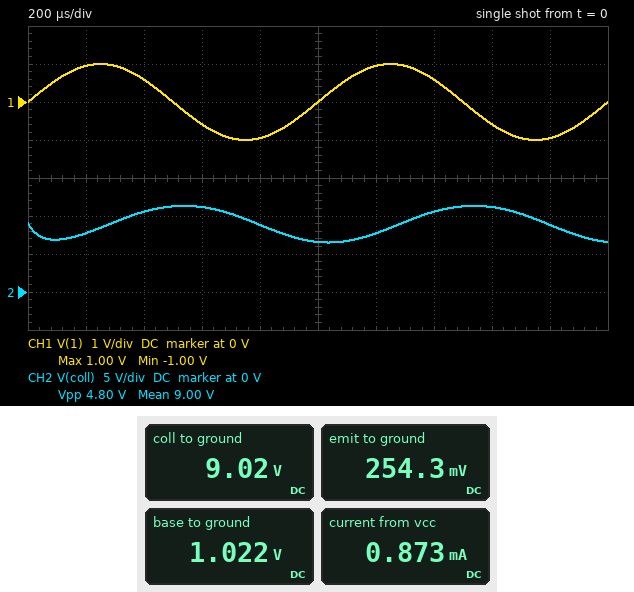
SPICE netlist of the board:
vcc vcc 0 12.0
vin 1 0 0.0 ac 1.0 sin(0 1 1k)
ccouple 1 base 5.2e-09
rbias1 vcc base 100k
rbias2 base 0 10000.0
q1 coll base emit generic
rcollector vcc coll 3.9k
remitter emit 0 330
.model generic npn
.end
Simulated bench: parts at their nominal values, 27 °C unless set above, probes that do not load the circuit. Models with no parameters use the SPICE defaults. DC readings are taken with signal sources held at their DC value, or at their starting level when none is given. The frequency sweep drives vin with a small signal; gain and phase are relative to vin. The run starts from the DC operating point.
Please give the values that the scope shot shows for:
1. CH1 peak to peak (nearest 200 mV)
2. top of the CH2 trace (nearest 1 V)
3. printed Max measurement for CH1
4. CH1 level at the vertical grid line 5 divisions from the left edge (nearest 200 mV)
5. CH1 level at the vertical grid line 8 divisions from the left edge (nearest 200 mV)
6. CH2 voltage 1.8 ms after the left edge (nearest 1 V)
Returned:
2.0 V
11 V
1.00 V
0 V
-600 mV
9 V
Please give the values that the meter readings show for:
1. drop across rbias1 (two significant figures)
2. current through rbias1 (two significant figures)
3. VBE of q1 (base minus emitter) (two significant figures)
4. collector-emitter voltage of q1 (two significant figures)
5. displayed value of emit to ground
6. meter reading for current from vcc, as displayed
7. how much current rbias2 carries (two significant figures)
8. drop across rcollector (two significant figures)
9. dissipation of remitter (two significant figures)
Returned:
11 V
110 µA
770 mV
8.8 V
254.3 mV
0.873 mA
100 µA
3.0 V
200 µW
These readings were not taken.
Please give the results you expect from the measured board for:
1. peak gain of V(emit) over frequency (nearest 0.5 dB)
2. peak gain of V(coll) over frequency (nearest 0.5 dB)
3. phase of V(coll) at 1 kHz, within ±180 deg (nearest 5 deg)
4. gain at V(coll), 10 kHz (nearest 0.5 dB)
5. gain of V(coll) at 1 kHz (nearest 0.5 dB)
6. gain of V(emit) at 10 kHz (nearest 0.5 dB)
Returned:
-1.0 dB
20.5 dB
-105 deg
20.0 dB
8.0 dB
-1.5 dB
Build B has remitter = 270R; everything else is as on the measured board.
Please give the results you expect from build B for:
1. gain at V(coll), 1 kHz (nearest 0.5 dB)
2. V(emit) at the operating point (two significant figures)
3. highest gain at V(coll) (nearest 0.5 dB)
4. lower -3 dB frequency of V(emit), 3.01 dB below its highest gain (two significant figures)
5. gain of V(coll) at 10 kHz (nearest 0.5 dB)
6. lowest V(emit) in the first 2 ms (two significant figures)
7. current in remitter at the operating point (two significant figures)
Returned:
9.0 dB
240 mV
22.0 dB
4.4 kHz
21.5 dB
53 mV
890 µA
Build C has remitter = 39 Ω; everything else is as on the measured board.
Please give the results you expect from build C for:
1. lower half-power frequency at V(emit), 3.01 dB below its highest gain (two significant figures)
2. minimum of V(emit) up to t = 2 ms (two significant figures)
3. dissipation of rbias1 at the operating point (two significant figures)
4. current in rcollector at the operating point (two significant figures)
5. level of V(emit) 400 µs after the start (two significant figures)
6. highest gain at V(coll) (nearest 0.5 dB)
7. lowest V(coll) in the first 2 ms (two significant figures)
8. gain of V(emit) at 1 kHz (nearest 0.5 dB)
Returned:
9.4 kHz
15 mV
1.2 mW
2.3 mA
32 mV
37.5 dB
250 mV
-21.5 dB
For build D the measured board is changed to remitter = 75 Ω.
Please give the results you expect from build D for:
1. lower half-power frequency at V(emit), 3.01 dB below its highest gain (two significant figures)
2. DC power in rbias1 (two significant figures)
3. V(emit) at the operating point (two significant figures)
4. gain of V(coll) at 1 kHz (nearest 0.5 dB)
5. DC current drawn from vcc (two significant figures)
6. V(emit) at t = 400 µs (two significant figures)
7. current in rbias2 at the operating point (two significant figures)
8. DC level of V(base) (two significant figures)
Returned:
6.8 kHz
1.2 mW
140 mV
16.0 dB
1.9 mA
54 mV
93 µA
930 mV
